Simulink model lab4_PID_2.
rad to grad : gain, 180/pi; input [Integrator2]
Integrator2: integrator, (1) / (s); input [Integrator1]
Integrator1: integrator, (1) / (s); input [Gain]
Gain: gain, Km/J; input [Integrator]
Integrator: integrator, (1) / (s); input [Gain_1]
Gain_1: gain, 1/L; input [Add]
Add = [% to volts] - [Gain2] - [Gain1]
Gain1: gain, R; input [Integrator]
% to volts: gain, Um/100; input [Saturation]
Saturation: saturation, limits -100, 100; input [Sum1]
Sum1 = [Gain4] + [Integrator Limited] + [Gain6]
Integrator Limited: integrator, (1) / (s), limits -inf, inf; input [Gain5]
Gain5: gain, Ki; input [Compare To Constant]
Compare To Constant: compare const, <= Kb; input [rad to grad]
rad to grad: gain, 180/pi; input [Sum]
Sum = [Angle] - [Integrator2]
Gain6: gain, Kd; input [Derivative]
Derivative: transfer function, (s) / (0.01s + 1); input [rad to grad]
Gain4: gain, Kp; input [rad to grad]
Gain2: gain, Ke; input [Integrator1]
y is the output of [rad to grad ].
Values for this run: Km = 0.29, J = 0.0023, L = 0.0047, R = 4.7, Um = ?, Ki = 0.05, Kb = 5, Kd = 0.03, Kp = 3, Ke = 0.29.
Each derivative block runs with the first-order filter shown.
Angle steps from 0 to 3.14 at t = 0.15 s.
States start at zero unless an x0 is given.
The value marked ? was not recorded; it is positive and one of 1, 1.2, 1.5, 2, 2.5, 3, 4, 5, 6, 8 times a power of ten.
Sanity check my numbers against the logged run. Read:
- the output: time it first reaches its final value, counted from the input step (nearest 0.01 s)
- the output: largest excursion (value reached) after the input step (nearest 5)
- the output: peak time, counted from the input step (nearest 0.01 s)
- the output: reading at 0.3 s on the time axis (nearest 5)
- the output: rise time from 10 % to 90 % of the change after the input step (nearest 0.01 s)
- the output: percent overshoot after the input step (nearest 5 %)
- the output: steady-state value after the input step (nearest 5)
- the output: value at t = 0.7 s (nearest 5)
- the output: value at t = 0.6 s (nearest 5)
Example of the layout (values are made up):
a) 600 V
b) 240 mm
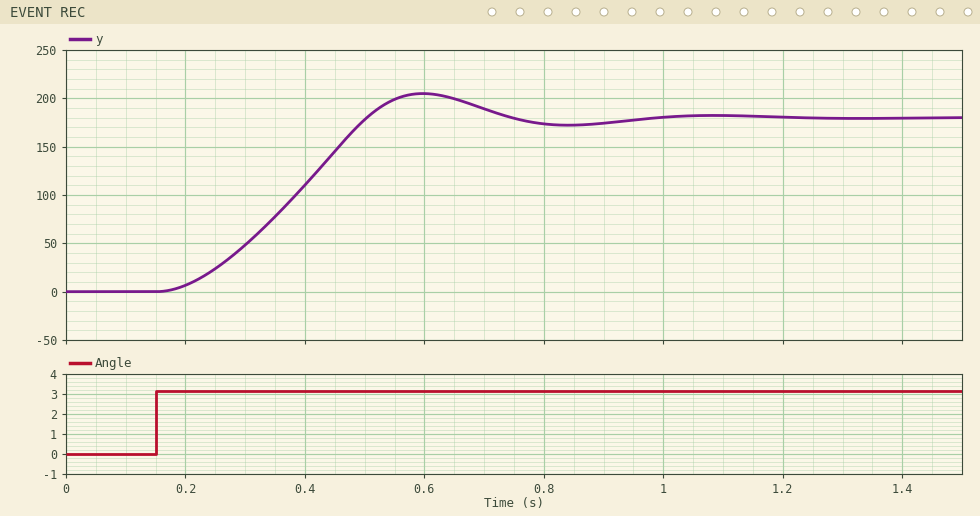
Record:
a) 0.35 s
b) 205
c) 0.45 s
d) 50
e) 0.24 s
f) 15 %
g) 180
h) 190
i) 205
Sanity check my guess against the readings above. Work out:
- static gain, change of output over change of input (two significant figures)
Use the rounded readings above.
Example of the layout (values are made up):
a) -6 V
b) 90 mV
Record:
a) 57
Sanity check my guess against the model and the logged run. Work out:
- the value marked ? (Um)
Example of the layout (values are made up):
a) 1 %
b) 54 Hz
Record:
a) 4
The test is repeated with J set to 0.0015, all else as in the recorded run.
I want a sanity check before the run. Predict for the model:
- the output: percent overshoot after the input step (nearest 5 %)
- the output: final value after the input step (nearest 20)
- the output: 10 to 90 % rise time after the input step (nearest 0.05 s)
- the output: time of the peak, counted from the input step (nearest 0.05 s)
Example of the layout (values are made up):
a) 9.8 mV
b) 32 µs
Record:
a) 10 %
b) 180
c) 0.20 s
d) 0.40 s
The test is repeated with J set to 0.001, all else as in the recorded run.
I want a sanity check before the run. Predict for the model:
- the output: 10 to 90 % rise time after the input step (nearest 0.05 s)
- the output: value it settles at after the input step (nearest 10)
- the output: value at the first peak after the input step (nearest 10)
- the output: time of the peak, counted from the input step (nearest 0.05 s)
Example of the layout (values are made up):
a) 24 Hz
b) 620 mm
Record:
a) 0.20 s
b) 180
c) 190
d) 0.35 s
